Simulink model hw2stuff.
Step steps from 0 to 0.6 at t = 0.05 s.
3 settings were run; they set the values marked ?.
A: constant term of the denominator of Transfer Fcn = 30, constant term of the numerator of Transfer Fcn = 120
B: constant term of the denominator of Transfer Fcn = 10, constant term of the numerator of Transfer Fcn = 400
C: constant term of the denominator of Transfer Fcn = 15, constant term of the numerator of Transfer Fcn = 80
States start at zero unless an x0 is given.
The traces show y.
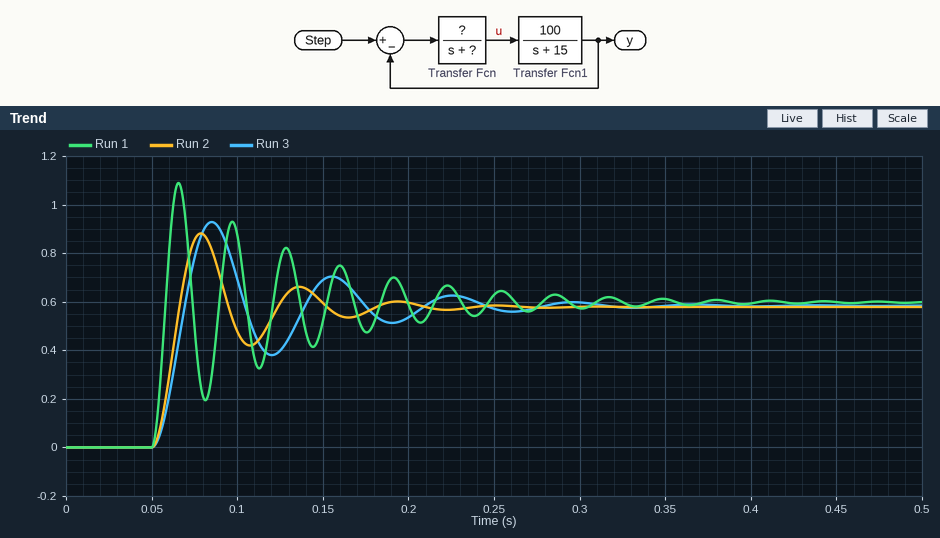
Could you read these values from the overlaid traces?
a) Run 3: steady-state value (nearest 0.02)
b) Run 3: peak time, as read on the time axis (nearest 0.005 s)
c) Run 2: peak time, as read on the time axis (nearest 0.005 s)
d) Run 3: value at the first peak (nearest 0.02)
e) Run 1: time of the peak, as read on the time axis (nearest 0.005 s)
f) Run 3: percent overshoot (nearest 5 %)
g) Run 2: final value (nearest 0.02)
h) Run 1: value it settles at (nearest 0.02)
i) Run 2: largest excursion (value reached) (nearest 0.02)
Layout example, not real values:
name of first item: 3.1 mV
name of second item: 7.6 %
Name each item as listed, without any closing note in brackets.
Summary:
Run 3: steady-state value: 0.58
Run 3: peak time, as read on the time axis: 0.085 s
Run 2: peak time, as read on the time axis: 0.080 s
Run 3: value at the first peak: 0.92
Run 1: time of the peak, as read on the time axis: 0.065 s
Run 3: percent overshoot: 60 %
Run 2: final value: 0.58
Run 1: value it settles at: 0.60
Run 2: largest excursion (value reached): 0.88
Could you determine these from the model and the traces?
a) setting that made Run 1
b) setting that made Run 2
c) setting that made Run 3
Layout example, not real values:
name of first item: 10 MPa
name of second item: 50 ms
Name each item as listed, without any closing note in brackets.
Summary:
setting that made Run 1: B
setting that made Run 2: A
setting that made Run 3: C
